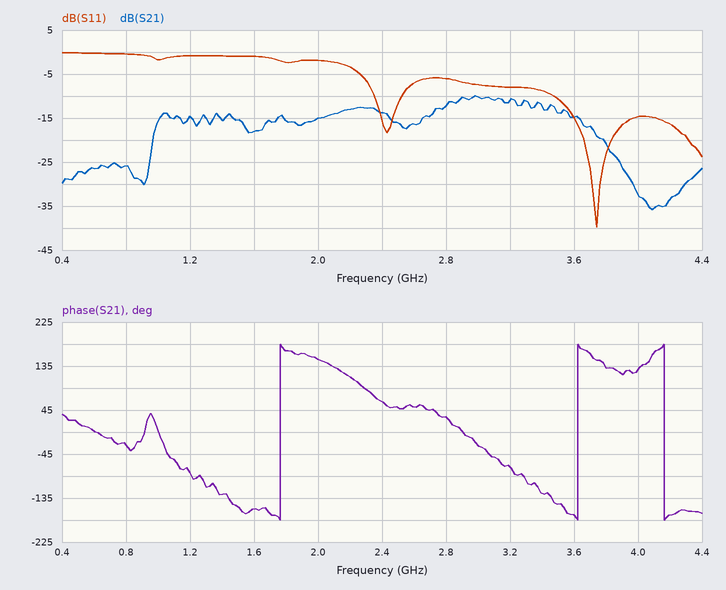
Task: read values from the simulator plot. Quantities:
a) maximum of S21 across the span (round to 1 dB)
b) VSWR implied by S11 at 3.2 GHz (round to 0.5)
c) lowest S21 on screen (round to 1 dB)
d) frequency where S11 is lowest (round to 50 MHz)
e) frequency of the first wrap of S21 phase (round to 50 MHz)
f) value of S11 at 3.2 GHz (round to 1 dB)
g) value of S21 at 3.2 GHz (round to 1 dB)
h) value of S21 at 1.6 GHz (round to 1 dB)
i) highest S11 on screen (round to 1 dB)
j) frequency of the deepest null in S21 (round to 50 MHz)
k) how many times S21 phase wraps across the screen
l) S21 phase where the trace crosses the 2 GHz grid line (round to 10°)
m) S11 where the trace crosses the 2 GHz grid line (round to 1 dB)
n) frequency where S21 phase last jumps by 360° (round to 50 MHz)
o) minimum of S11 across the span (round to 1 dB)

-10 dB
2.5
-36 dB
3.75 GHz
1.75 GHz
-8 dB
-11 dB
-18 dB
0 dB
4.10 GHz
3
150°
-2 dB
4.15 GHz
-40 dB
